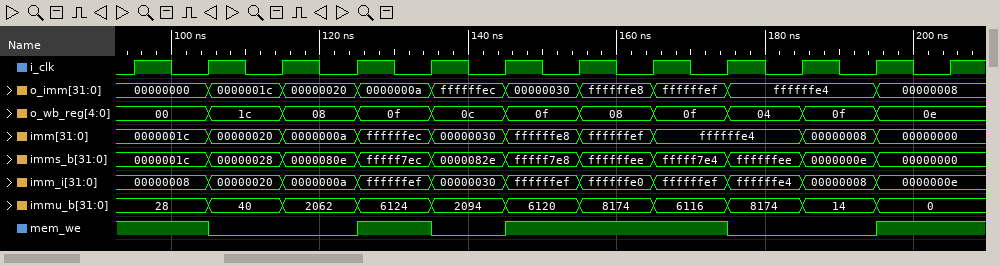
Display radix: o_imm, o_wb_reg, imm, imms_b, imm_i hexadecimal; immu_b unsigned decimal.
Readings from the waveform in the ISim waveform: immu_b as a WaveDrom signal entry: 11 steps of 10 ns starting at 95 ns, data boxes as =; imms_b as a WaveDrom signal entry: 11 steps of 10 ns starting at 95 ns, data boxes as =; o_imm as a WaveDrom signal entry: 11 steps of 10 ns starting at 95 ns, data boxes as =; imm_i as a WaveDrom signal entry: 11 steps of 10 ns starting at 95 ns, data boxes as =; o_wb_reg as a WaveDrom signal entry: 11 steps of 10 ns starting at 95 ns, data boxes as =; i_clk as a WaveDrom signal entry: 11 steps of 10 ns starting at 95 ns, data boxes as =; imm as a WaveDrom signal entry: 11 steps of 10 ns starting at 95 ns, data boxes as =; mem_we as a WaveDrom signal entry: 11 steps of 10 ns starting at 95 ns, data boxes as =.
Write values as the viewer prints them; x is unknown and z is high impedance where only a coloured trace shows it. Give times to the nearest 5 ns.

{name: 'immu_b', wave: '===========', data: '28 40 2062 6124 2094 6120 8174 6116 8174 14 0'}
{name: 'imms_b', wave: '===========', data: '0000001c 00000028 0000080e fffff7ec 0000082e fffff7e8 ffffffee fffff7e4 ffffffee 0000000e 00000000'}
{name: 'o_imm', wave: '=========.=', data: '00000000 0000001c 00000020 0000000a ffffffec 00000030 ffffffe8 ffffffef ffffffe4 00000008'}
{name: 'imm_i', wave: '===========', data: '00000008 00000020 0000000a ffffffef 00000030 ffffffef ffffffe0 ffffffef ffffffe4 00000008 0000000e'}
{name: 'o_wb_reg', wave: '===========', data: '00 1c 08 0f 0c 0f 08 0f 04 0f 0e'}
{name: 'i_clk', wave: 'p..........'}
{name: 'imm', wave: '========.==', data: '0000001c 00000020 0000000a ffffffec 00000030 ffffffe8 ffffffef ffffffe4 00000008 00000000'}
{name: 'mem_we', wave: '10.101..0.1'}
